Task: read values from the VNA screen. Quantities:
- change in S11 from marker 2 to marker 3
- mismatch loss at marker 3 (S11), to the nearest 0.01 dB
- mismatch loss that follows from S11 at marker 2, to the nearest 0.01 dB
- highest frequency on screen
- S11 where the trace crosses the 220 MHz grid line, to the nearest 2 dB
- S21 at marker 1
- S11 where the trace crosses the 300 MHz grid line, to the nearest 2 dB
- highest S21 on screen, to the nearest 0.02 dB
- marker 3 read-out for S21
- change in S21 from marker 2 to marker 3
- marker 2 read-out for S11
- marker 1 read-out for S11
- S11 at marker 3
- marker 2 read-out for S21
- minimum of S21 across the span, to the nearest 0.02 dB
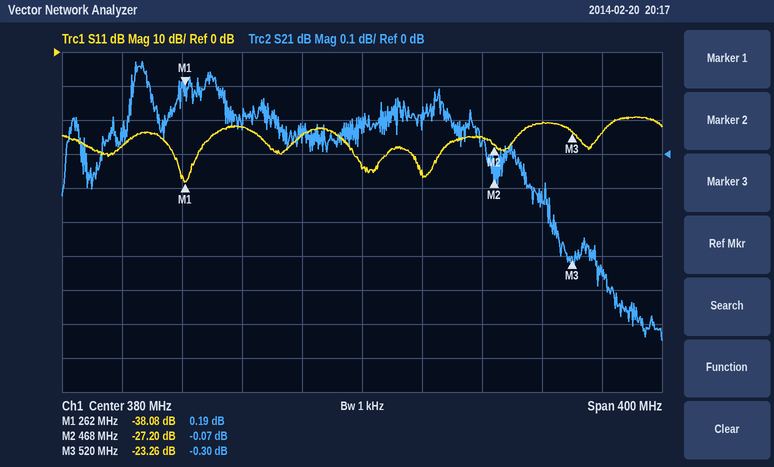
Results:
3.94 dB
0.02 dB
0.01 dB
580 MHz
-28 dB
0.19 dB
-22 dB
0.28 dB
-0.30 dB
-0.23 dB
-27.20 dB
-38.08 dB
-23.26 dB
-0.07 dB
-0.54 dB
